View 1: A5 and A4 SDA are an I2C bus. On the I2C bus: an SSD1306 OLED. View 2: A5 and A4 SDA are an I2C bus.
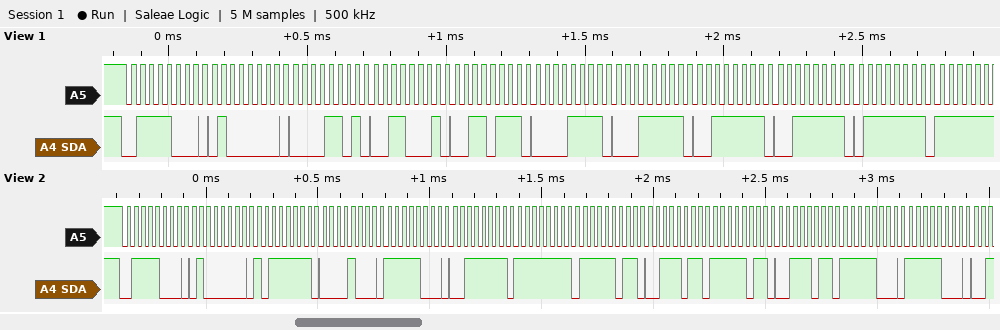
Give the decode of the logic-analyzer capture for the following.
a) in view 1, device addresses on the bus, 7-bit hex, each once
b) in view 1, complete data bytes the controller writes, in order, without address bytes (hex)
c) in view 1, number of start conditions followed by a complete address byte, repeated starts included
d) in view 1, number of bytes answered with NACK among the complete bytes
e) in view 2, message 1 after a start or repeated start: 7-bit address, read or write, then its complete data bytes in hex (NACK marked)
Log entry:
0x3C
40 0D 31 37 0F 1F 3F 3F 7F
1
0
0x3C write: 40 BF 08 F8 3F FF FB 3B FB 3B F8 F8
